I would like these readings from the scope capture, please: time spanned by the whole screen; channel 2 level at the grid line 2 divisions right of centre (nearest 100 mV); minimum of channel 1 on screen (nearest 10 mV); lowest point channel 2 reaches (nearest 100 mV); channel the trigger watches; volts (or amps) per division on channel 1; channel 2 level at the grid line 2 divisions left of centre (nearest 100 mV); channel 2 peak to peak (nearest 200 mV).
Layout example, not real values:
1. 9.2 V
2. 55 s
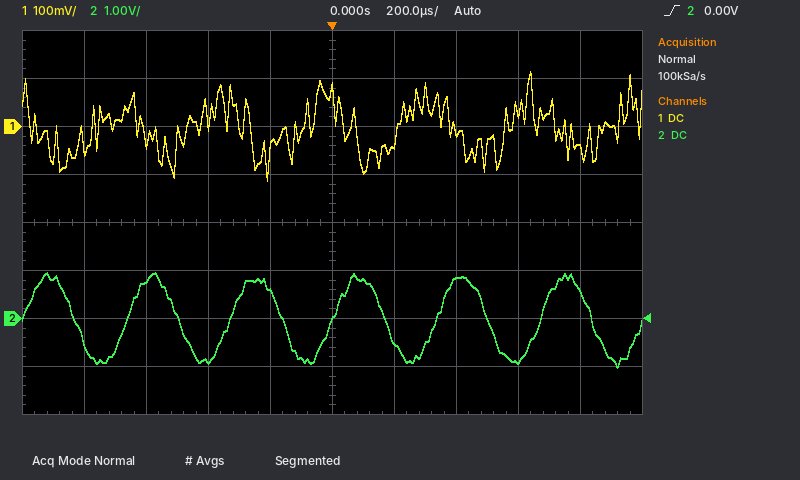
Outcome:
1. 2 ms
2. 800 mV
3. -110 mV
4. -1.0 V
5. channel 2
6. 100 mV
7. -900 mV
8. 2.0 V
